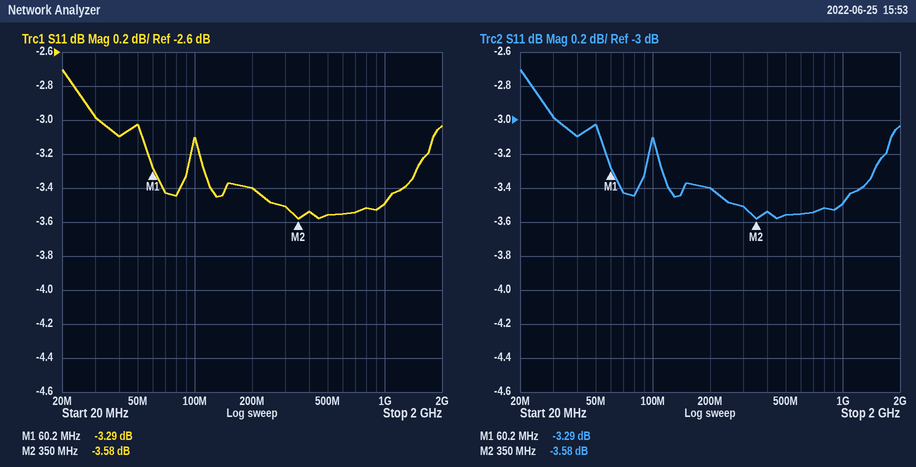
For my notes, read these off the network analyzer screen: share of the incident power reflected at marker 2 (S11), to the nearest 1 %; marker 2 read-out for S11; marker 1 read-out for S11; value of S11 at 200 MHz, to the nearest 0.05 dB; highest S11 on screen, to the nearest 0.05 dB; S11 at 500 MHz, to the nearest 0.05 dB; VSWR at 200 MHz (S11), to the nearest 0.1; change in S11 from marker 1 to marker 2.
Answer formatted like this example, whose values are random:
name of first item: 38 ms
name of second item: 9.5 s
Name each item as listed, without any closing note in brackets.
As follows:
share of the incident power reflected at marker 2 (S11), to the nearest 1 %: 44 %
marker 2 read-out for S11: -3.58 dB
marker 1 read-out for S11: -3.29 dB
value of S11 at 200 MHz, to the nearest 0.05 dB: -3.40 dB
highest S11 on screen, to the nearest 0.05 dB: -2.70 dB
S11 at 500 MHz, to the nearest 0.05 dB: -3.55 dB
VSWR at 200 MHz (S11), to the nearest 0.1: 5.2
change in S11 from marker 1 to marker 2: -0.29 dB
